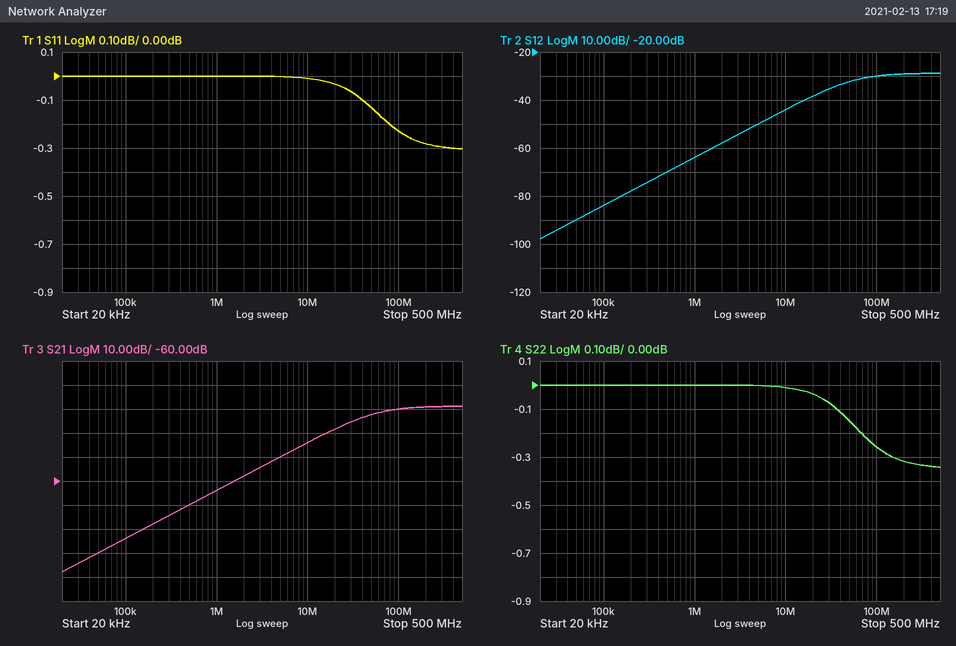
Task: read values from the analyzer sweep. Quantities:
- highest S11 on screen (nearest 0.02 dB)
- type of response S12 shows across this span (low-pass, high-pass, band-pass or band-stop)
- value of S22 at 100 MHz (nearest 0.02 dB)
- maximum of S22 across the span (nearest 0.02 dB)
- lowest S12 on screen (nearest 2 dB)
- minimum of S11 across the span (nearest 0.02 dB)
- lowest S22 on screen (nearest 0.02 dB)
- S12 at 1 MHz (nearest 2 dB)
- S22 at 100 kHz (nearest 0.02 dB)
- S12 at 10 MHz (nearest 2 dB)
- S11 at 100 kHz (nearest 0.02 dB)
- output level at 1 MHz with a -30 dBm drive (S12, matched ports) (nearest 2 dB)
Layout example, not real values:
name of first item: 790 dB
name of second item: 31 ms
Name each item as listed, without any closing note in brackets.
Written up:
highest S11 on screen: 0.00 dB
type of response S12 shows across this span: high-pass
value of S22 at 100 MHz: -0.26 dB
maximum of S22 across the span: 0.00 dB
lowest S12 on screen: -98 dB
minimum of S11 across the span: -0.30 dB
lowest S22 on screen: -0.34 dB
S12 at 1 MHz: -64 dB
S22 at 100 kHz: 0.00 dB
S12 at 10 MHz: -44 dB
S11 at 100 kHz: 0.00 dB
output level at 1 MHz with a -30 dBm drive (S12, matched ports): -94 dBm
